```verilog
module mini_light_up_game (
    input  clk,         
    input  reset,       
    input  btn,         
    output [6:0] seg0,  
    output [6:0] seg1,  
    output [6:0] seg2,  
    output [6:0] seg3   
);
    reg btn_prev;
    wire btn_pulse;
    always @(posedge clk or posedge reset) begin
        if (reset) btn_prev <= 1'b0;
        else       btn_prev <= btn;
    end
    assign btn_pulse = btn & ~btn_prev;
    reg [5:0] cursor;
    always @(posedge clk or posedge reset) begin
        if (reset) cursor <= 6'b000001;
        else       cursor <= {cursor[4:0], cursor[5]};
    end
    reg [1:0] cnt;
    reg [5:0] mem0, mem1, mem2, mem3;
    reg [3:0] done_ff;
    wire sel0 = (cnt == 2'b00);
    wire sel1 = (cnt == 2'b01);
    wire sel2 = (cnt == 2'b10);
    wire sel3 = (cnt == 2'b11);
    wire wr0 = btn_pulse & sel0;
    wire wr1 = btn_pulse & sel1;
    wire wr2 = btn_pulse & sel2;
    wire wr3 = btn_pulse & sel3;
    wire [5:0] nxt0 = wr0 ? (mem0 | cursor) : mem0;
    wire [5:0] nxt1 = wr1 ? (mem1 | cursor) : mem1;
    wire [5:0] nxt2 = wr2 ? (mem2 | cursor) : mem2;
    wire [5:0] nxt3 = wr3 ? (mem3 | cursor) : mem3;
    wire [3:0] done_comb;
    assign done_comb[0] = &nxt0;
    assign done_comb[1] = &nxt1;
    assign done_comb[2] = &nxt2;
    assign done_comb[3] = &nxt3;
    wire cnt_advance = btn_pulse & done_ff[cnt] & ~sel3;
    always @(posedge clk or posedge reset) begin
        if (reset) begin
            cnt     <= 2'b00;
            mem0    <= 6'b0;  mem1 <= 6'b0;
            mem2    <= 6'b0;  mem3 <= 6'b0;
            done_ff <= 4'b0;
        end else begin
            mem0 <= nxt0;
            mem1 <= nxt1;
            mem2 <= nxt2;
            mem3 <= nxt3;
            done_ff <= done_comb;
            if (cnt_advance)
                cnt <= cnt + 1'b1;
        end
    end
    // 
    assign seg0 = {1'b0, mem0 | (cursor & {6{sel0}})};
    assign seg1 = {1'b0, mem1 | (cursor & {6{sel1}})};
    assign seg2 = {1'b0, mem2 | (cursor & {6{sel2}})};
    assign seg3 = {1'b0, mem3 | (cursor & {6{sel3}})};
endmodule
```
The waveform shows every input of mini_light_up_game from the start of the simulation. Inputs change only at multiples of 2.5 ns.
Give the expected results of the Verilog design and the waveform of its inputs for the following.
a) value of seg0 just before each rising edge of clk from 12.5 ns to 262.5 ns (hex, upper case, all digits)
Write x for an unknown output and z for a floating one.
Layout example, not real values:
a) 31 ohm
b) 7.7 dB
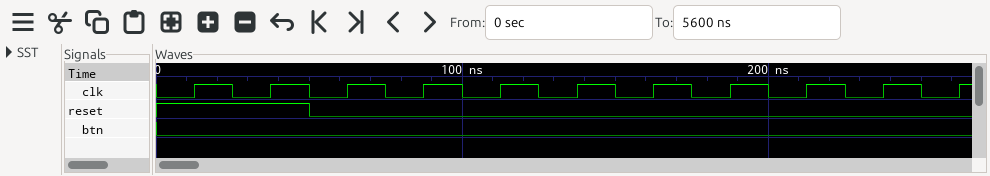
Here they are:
a) 01, 01, 01, 02, 04, 08, 10, 20, 01, 02, 04
